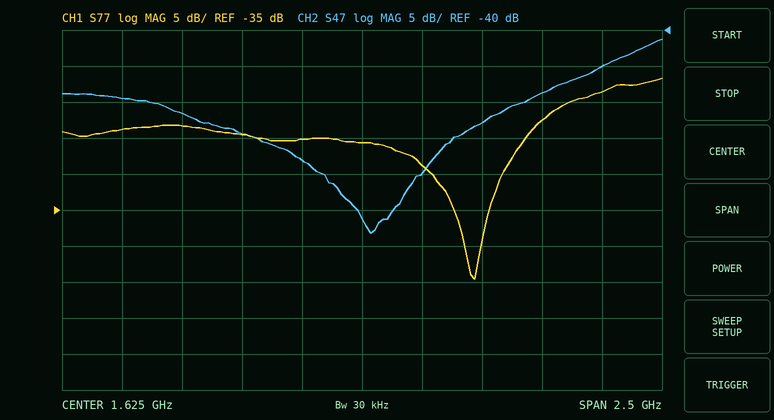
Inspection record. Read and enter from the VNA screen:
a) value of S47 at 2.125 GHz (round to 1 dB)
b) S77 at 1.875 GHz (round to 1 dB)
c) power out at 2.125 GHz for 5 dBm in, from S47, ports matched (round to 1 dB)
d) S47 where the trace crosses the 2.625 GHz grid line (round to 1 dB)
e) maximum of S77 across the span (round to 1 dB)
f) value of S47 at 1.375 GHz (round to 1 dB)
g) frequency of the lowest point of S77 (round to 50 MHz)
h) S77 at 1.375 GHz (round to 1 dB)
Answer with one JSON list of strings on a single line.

["-53 dB", "-29 dB", "-48 dBm", "-45 dB", "-17 dB", "-58 dB", "2.10 GHz", "-25 dB"]
